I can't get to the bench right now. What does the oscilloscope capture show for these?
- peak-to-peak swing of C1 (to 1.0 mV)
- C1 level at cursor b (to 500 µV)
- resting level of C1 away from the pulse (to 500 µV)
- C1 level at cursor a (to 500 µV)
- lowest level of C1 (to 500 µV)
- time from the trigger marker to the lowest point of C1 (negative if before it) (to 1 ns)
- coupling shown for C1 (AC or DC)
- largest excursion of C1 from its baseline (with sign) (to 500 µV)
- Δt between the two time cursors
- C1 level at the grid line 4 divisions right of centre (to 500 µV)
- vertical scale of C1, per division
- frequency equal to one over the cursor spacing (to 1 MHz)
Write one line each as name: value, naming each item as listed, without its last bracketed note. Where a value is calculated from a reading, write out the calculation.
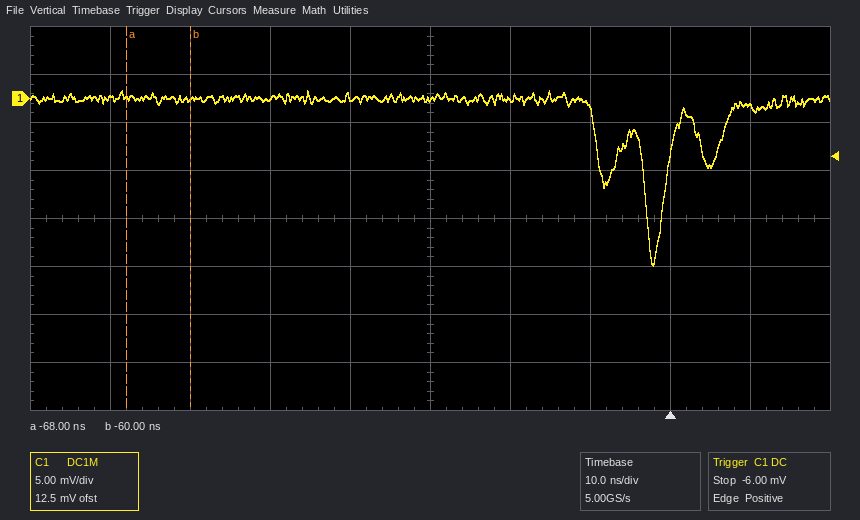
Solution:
peak-to-peak swing of C1: 18.0 mV
C1 level at cursor b: 0.0 mV
resting level of C1 away from the pulse: 0.0 mV
C1 level at cursor a: 0.0 mV
lowest level of C1: -17.5 mV
time from the trigger marker to the lowest point of C1 (negative if before it): -2 ns
coupling shown for C1: DC
largest excursion of C1 from its baseline (with sign): -17.5 mV − (0.0 mV) = -17.5 mV
Δt between the two time cursors: -60 ns − (-68 ns) = 8 ns
C1 level at the grid line 4 divisions right of centre: -1.0 mV
vertical scale of C1, per division: 5 mV
frequency equal to one over the cursor spacing: 1 / 8 ns ≈ 125 MHz
